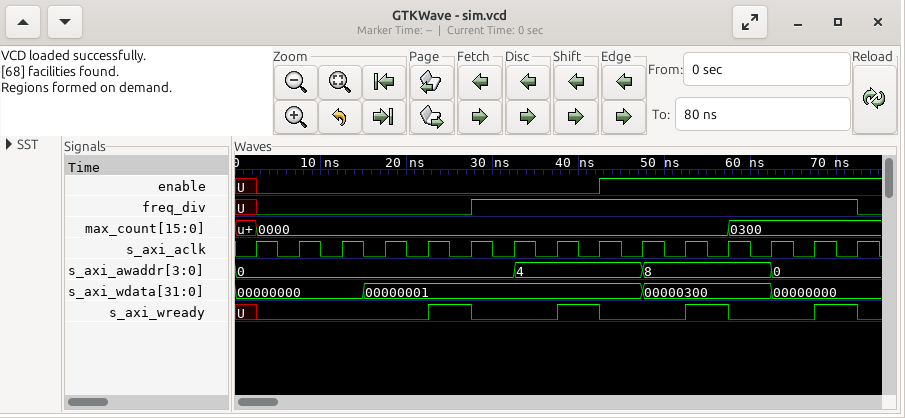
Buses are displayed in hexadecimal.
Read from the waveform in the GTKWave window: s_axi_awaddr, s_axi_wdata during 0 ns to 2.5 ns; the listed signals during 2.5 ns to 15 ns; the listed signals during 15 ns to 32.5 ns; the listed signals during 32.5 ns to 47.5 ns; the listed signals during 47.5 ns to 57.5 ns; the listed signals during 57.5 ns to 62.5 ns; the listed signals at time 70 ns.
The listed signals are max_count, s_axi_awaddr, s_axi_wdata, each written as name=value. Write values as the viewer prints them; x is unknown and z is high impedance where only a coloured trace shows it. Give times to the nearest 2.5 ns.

s_axi_awaddr=0, s_axi_wdata=00000000
max_count=0000, s_axi_awaddr=0, s_axi_wdata=00000000
max_count=0000, s_axi_awaddr=0, s_axi_wdata=00000001
max_count=0000, s_axi_awaddr=4, s_axi_wdata=00000001
max_count=0000, s_axi_awaddr=8, s_axi_wdata=00000300
max_count=0300, s_axi_awaddr=8, s_axi_wdata=00000300
max_count=0300, s_axi_awaddr=0, s_axi_wdata=00000000
